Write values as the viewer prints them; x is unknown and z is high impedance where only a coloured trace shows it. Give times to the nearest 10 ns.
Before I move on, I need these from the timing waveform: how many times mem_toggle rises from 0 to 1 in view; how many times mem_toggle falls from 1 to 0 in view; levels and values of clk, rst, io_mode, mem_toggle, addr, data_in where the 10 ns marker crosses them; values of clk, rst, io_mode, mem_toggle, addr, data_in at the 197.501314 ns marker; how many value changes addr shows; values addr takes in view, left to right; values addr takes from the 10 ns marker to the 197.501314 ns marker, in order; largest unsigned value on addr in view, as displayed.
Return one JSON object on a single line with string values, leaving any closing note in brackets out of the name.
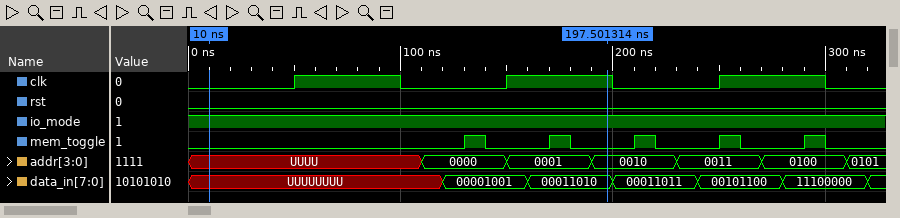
{"how many times mem_toggle rises from 0 to 1 in view": "5", "how many times mem_toggle falls from 1 to 0 in view": "5", "levels and values of clk, rst, io_mode, mem_toggle, addr, data_in where the 10 ns marker crosses them": "clk=0, rst=0, io_mode=1, mem_toggle=0, addr=UUUU, data_in=UUUUUUUU", "values of clk, rst, io_mode, mem_toggle, addr, data_in at the 197.501314 ns marker": "clk=1, rst=0, io_mode=1, mem_toggle=0, addr=0010, data_in=00011010", "how many value changes addr shows": "6", "values addr takes in view, left to right": "UUUU, 0000, 0001, 0010, 0011, 0100, 0101", "values addr takes from the 10 ns marker to the 197.501314 ns marker, in order": "UUUU, 0000, 0001, 0010", "largest unsigned value on addr in view, as displayed": "0101"}
